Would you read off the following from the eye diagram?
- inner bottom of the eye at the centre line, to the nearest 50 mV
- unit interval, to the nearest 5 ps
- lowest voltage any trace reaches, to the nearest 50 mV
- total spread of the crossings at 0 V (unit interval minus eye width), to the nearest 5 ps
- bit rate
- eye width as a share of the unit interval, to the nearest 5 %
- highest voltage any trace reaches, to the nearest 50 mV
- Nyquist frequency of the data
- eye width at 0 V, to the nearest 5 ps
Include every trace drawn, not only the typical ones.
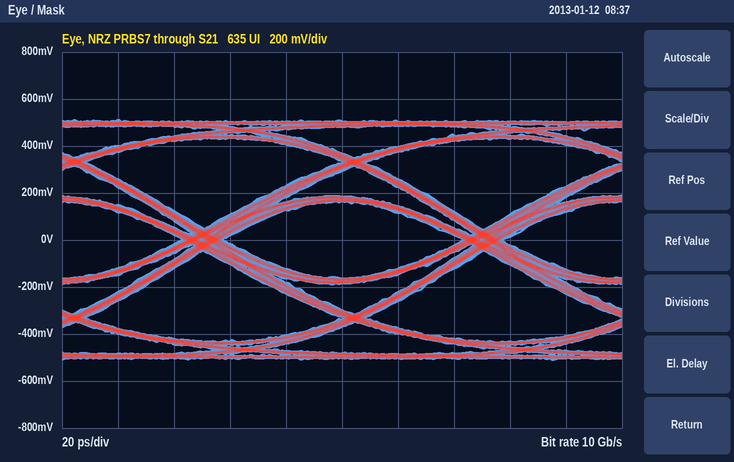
-150 mV
100 ps
-500 mV
15 ps
10 Gb/s
85 %
500 mV
5 GHz
85 ps
